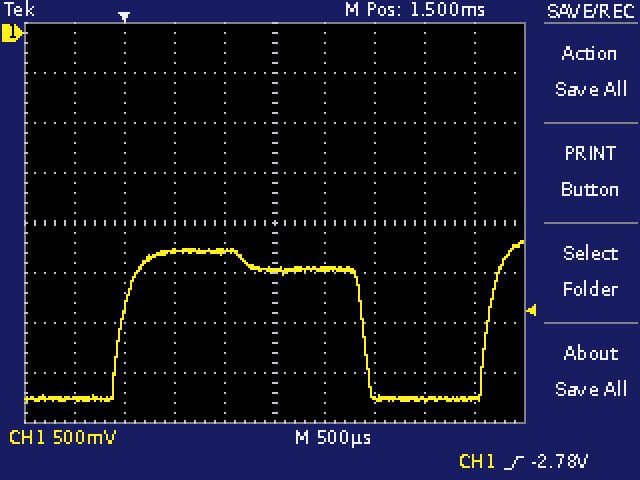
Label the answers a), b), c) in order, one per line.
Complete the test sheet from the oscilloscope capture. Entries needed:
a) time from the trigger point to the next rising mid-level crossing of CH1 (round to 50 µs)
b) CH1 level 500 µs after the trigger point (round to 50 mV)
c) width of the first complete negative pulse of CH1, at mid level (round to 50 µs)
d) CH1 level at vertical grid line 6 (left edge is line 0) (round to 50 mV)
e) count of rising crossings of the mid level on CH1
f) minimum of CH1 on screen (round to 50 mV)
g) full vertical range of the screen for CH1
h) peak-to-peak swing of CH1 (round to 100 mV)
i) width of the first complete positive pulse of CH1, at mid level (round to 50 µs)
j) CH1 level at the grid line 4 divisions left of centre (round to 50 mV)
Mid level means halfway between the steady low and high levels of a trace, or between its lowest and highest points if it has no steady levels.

a) 3.65 ms
b) -2.20 V
c) 1.25 ms
d) -2.35 V
e) 2
f) -3.70 V
g) 4 V
h) 1.60 V
i) 2.40 ms
j) -3.65 V
